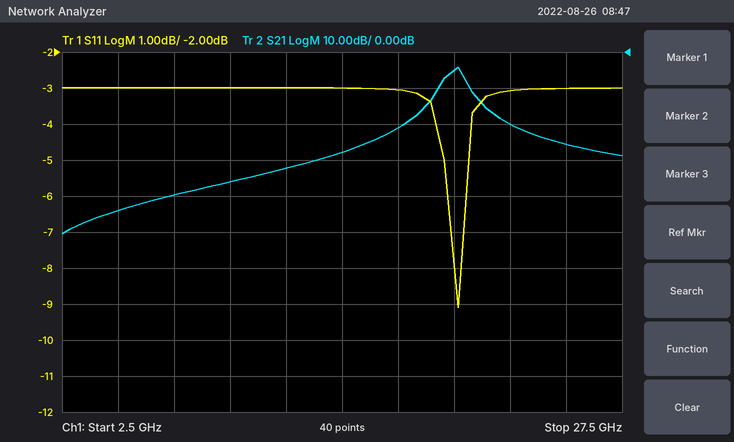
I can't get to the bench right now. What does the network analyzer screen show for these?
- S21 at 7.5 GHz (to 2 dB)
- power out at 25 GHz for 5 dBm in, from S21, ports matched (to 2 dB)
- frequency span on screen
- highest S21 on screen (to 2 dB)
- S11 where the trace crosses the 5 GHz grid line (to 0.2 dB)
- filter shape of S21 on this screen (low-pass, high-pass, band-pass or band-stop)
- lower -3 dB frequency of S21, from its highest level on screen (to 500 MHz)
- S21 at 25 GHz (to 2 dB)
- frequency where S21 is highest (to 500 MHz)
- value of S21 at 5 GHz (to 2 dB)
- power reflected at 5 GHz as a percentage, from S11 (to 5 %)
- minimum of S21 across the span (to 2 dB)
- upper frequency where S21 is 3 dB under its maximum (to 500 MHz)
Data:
-40 dB
-20 dBm
25 GHz
-4 dB
-3.0 dB
band-pass
19.5 GHz
-26 dB
20.0 GHz
-44 dB
50 %
-50 dB
20.5 GHz
